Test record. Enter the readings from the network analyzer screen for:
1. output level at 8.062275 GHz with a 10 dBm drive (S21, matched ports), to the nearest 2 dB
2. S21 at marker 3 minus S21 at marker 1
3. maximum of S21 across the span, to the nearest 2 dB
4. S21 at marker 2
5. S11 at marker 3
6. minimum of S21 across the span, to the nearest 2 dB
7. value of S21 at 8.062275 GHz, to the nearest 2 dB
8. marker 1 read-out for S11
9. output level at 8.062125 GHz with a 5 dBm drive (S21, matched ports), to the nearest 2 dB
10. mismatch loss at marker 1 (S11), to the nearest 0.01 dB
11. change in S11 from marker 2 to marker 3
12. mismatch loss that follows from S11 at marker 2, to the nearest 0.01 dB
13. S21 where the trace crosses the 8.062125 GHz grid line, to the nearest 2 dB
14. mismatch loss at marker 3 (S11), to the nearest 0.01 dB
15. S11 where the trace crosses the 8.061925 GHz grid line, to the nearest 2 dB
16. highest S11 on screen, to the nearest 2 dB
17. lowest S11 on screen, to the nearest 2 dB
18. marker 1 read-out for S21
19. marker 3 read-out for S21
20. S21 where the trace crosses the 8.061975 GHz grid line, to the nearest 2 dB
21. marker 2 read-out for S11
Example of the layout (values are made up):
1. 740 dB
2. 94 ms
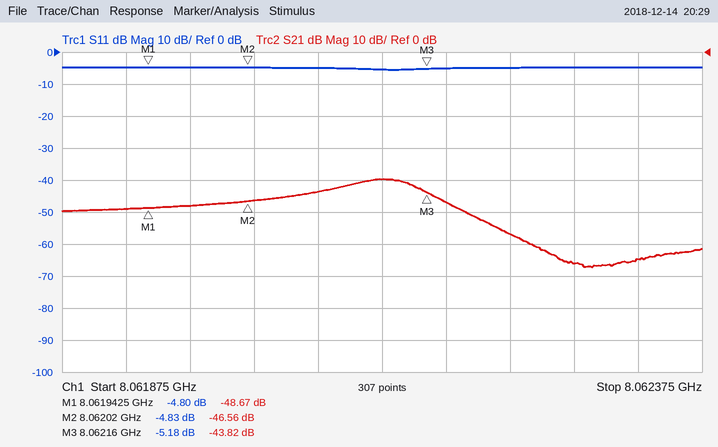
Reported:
1. -56 dBm
2. 4.85 dB
3. -40 dB
4. -46.56 dB
5. -5.18 dB
6. -68 dB
7. -66 dB
8. -4.80 dB
9. -34 dBm
10. 1.75 dB
11. -0.35 dB
12. 1.73 dB
13. -40 dB
14. 1.57 dB
15. -4 dB
16. -4 dB
17. -6 dB
18. -48.67 dB
19. -43.82 dB
20. -48 dB
21. -4.83 dB
